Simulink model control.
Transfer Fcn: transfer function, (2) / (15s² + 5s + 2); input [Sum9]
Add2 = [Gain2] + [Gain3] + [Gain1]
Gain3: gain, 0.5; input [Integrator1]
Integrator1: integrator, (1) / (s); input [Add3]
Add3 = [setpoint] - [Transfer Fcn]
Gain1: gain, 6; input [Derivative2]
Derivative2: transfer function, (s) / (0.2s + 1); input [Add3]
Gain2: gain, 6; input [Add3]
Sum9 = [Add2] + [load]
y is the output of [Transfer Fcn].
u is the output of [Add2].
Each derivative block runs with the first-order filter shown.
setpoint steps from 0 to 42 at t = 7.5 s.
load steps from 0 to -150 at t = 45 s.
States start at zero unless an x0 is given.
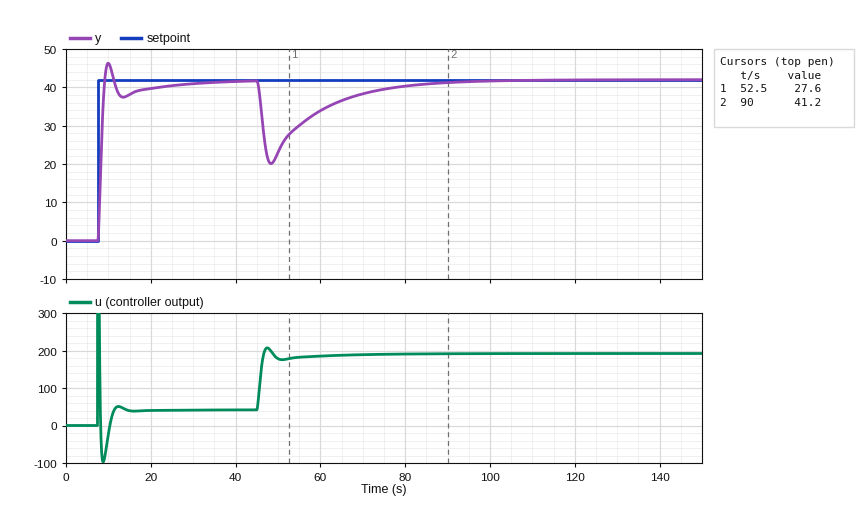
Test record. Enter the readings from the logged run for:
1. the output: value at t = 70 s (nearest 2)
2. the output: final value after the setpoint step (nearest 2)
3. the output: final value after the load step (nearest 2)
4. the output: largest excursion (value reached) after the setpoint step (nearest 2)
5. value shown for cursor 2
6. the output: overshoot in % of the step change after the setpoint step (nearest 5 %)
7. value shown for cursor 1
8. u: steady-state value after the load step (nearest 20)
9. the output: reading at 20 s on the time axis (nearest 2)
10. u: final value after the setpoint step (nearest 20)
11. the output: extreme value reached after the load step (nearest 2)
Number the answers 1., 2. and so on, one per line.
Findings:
1. 38
2. 42
3. 42
4. 46
5. 41.2
6. 10 %
7. 27.6
8. 200
9. 40
10. 40
11. 20
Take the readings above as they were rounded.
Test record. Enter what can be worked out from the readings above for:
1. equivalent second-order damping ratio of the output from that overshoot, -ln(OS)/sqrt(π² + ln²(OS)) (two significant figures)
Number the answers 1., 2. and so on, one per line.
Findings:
1. 0.59
